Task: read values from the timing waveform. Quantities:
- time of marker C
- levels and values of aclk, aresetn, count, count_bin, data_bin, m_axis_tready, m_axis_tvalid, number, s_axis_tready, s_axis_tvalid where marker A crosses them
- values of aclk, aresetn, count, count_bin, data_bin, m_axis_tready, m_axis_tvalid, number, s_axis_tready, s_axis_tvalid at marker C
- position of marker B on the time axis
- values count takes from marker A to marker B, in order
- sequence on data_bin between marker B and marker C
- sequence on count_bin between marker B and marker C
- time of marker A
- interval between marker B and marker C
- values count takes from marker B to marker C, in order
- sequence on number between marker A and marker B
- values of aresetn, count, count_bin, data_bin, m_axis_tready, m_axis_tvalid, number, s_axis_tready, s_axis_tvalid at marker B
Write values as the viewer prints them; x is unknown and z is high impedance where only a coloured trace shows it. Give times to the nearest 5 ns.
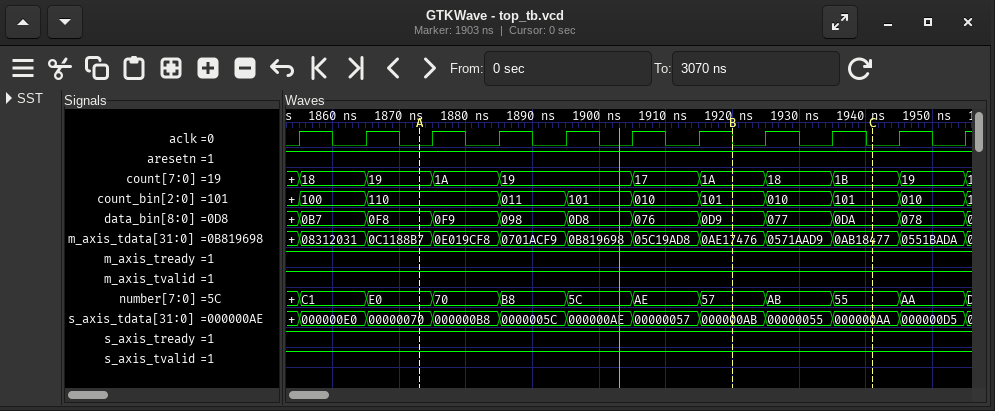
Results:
1940 ns
aclk=0, aresetn=1, count=19, count_bin=110, data_bin=0F8, m_axis_tready=1, m_axis_tvalid=1, number=E0, s_axis_tready=1, s_axis_tvalid=1
aclk=0, aresetn=1, count=1B, count_bin=101, data_bin=0DA, m_axis_tready=1, m_axis_tvalid=1, number=55, s_axis_tready=1, s_axis_tvalid=1
1920 ns
19, 1A, 19, 17, 1A
0D9, 077, 0DA
101, 010, 101
1875 ns
20 ns
1A, 18, 1B
E0, 70, B8, 5C, AE, 57
aresetn=1, count=1A, count_bin=101, data_bin=0D9, m_axis_tready=1, m_axis_tvalid=1, number=57, s_axis_tready=1, s_axis_tvalid=1
